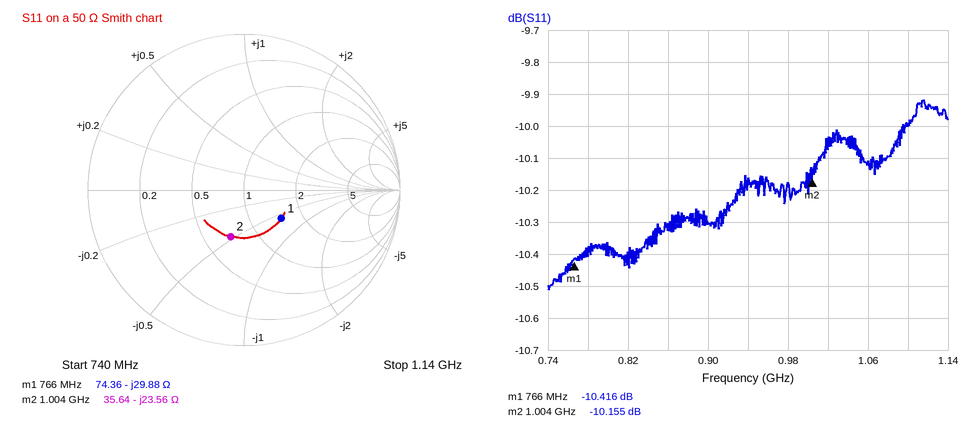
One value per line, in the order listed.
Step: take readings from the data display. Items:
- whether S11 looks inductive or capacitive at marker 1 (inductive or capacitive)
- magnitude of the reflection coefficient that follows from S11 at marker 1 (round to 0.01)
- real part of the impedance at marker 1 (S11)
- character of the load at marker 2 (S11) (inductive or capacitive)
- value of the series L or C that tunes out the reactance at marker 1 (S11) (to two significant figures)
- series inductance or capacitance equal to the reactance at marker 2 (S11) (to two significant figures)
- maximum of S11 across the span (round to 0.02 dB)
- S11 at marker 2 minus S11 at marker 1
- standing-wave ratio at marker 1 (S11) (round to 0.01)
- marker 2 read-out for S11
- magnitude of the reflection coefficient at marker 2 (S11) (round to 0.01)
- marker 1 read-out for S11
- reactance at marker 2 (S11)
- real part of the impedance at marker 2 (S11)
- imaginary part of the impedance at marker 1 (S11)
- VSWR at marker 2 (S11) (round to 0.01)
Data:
capacitive
0.30
74.36 Ω
capacitive
6.2 nH
6.7 pF
-9.92 dB
0.261 dB
1.86
-10.155 dB
0.31
-10.416 dB
-23.56 Ω
35.64 Ω
-29.88 Ω
1.90
